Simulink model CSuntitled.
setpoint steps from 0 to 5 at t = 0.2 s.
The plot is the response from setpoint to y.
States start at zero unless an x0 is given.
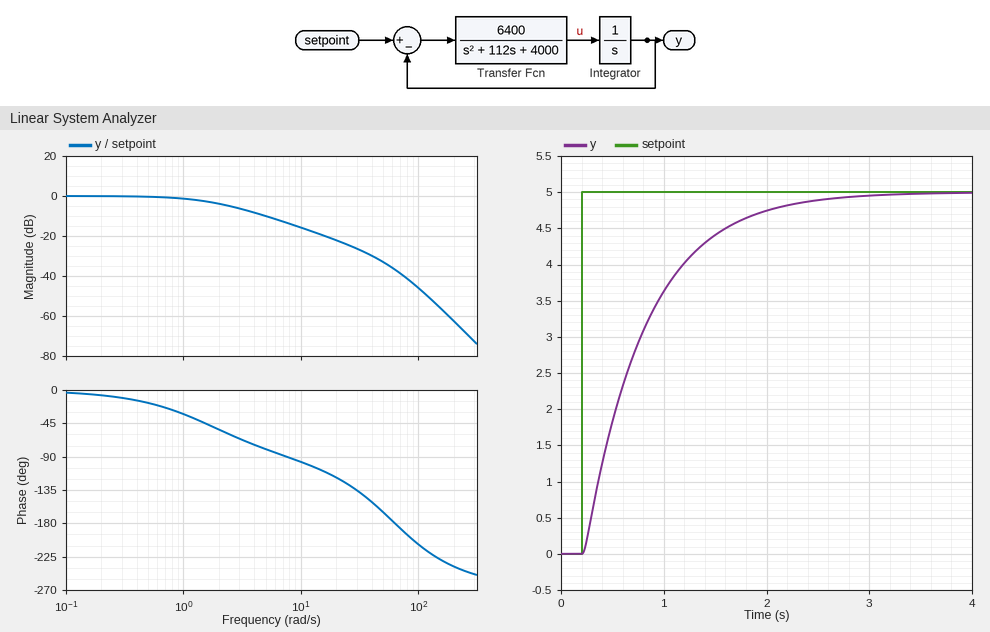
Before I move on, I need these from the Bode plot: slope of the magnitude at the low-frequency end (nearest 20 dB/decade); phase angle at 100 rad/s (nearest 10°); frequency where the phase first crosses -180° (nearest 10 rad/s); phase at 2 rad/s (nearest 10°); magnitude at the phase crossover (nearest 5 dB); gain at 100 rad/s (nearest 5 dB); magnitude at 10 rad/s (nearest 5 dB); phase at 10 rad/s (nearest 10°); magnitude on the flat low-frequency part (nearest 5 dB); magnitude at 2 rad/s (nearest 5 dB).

0 dB/decade
-210°
60 rad/s
-50°
-35 dB
-45 dB
-15 dB
-100°
0 dB
-5 dB
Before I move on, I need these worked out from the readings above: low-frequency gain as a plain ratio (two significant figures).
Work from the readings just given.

1.0
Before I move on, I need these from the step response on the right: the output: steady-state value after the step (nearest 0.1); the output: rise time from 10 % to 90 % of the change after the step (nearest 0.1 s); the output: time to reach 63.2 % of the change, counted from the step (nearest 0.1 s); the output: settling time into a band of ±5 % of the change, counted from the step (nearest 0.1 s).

5.0
1.3 s
0.6 s
1.8 s
